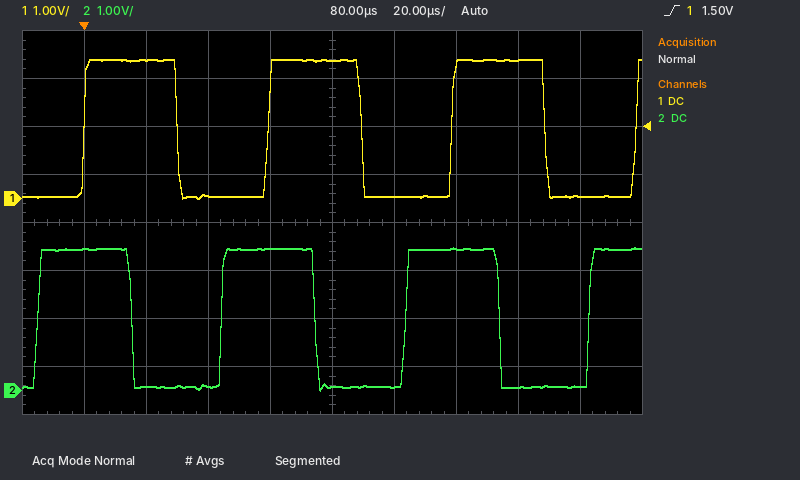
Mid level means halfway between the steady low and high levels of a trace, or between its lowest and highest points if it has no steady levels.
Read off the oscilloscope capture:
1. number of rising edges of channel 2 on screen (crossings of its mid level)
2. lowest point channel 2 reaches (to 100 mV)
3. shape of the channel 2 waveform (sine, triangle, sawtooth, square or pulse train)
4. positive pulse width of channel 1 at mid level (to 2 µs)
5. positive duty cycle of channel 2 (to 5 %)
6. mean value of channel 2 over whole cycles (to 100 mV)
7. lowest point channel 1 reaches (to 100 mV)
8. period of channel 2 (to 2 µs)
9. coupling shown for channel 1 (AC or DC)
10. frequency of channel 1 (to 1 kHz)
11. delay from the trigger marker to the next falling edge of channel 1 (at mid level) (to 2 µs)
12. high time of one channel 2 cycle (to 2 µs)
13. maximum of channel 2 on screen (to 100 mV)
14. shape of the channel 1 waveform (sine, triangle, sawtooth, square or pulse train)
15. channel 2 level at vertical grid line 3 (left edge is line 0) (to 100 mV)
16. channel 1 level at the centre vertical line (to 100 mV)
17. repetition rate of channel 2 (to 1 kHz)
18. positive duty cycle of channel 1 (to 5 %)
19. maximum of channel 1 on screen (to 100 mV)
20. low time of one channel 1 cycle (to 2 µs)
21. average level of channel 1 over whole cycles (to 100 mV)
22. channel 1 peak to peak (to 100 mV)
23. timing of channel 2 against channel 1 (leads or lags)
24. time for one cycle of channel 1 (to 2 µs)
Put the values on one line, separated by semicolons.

4; 0.0 V; square; 30 µs; 50 %; 1.5 V; 0.0 V; 60 µs; DC; 17 kHz; 30 µs; 30 µs; 3.0 V; square; 100 mV; 2.9 V; 17 kHz; 50 %; 2.9 V; 30 µs; 1.5 V; 2.9 V; leads; 60 µs
